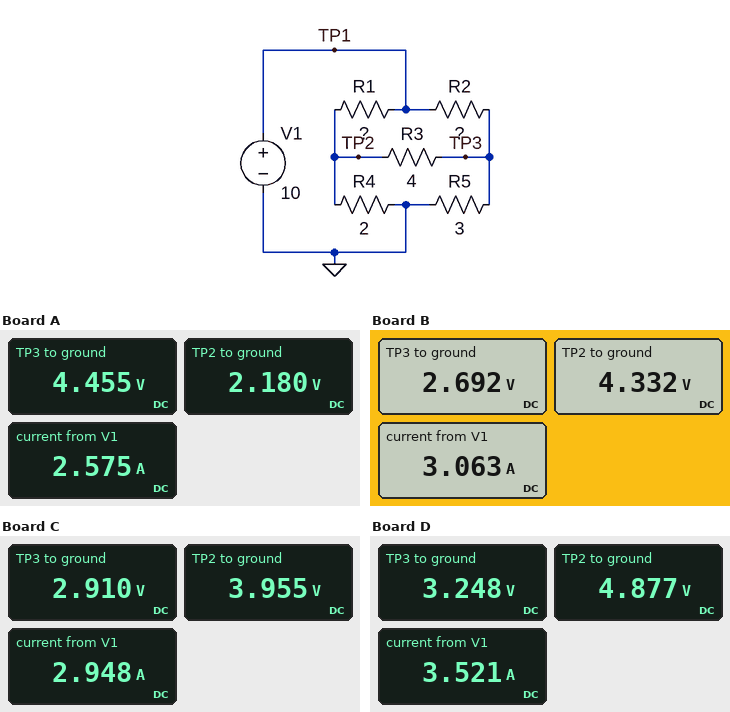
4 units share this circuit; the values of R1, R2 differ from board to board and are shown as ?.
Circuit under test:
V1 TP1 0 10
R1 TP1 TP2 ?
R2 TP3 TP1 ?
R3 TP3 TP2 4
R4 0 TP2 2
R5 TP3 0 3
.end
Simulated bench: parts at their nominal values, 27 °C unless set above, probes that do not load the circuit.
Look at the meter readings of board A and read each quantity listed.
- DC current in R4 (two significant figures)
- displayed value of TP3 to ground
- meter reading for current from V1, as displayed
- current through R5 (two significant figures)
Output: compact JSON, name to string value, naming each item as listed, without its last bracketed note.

{"DC current in R4": "1.1 A", "displayed value of TP3 to ground": "4.455 V", "meter reading for current from V1, as displayed": "2.575 A", "current through R5": "1.5 A"}
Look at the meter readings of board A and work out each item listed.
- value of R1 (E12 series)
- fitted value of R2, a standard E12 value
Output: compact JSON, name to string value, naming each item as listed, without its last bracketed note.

{"value of R1": "15 Ω", "fitted value of R2, a standard E12 value": "2.7 Ω"}
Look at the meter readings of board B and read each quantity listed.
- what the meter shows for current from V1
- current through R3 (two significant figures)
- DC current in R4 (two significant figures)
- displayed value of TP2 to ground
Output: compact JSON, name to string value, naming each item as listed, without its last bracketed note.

{"what the meter shows for current from V1": "3.063 A", "current through R3": "410 mA", "DC current in R4": "2.2 A", "displayed value of TP2 to ground": "4.332 V"}
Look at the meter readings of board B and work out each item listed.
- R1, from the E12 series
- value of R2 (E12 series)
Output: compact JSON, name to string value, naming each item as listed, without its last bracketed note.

{"R1, from the E12 series": "2.2 Ω", "value of R2": "15 Ω"}
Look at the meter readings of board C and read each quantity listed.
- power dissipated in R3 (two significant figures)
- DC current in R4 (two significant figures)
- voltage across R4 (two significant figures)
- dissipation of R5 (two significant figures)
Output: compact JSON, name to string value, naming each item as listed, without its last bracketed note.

{"power dissipated in R3": "270 mW", "DC current in R4": "2.0 A", "voltage across R4": "4.0 V", "dissipation of R5": "2.8 W"}
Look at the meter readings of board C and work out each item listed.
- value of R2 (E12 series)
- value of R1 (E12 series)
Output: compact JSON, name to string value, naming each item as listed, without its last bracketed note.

{"value of R2": "10 Ω", "value of R1": "2.7 Ω"}
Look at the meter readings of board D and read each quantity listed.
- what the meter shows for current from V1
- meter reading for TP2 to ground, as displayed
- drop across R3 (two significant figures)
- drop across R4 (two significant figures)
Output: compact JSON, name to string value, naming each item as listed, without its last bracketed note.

{"what the meter shows for current from V1": "3.521 A", "meter reading for TP2 to ground, as displayed": "4.877 V", "drop across R3": "1.6 V", "drop across R4": "4.9 V"}
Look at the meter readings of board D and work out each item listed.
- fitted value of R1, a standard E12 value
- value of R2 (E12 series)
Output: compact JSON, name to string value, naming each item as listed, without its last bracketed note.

{"fitted value of R1, a standard E12 value": "1.8 Ω", "value of R2": "10 Ω"}
